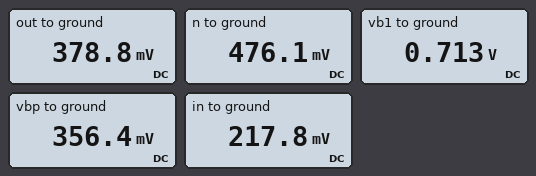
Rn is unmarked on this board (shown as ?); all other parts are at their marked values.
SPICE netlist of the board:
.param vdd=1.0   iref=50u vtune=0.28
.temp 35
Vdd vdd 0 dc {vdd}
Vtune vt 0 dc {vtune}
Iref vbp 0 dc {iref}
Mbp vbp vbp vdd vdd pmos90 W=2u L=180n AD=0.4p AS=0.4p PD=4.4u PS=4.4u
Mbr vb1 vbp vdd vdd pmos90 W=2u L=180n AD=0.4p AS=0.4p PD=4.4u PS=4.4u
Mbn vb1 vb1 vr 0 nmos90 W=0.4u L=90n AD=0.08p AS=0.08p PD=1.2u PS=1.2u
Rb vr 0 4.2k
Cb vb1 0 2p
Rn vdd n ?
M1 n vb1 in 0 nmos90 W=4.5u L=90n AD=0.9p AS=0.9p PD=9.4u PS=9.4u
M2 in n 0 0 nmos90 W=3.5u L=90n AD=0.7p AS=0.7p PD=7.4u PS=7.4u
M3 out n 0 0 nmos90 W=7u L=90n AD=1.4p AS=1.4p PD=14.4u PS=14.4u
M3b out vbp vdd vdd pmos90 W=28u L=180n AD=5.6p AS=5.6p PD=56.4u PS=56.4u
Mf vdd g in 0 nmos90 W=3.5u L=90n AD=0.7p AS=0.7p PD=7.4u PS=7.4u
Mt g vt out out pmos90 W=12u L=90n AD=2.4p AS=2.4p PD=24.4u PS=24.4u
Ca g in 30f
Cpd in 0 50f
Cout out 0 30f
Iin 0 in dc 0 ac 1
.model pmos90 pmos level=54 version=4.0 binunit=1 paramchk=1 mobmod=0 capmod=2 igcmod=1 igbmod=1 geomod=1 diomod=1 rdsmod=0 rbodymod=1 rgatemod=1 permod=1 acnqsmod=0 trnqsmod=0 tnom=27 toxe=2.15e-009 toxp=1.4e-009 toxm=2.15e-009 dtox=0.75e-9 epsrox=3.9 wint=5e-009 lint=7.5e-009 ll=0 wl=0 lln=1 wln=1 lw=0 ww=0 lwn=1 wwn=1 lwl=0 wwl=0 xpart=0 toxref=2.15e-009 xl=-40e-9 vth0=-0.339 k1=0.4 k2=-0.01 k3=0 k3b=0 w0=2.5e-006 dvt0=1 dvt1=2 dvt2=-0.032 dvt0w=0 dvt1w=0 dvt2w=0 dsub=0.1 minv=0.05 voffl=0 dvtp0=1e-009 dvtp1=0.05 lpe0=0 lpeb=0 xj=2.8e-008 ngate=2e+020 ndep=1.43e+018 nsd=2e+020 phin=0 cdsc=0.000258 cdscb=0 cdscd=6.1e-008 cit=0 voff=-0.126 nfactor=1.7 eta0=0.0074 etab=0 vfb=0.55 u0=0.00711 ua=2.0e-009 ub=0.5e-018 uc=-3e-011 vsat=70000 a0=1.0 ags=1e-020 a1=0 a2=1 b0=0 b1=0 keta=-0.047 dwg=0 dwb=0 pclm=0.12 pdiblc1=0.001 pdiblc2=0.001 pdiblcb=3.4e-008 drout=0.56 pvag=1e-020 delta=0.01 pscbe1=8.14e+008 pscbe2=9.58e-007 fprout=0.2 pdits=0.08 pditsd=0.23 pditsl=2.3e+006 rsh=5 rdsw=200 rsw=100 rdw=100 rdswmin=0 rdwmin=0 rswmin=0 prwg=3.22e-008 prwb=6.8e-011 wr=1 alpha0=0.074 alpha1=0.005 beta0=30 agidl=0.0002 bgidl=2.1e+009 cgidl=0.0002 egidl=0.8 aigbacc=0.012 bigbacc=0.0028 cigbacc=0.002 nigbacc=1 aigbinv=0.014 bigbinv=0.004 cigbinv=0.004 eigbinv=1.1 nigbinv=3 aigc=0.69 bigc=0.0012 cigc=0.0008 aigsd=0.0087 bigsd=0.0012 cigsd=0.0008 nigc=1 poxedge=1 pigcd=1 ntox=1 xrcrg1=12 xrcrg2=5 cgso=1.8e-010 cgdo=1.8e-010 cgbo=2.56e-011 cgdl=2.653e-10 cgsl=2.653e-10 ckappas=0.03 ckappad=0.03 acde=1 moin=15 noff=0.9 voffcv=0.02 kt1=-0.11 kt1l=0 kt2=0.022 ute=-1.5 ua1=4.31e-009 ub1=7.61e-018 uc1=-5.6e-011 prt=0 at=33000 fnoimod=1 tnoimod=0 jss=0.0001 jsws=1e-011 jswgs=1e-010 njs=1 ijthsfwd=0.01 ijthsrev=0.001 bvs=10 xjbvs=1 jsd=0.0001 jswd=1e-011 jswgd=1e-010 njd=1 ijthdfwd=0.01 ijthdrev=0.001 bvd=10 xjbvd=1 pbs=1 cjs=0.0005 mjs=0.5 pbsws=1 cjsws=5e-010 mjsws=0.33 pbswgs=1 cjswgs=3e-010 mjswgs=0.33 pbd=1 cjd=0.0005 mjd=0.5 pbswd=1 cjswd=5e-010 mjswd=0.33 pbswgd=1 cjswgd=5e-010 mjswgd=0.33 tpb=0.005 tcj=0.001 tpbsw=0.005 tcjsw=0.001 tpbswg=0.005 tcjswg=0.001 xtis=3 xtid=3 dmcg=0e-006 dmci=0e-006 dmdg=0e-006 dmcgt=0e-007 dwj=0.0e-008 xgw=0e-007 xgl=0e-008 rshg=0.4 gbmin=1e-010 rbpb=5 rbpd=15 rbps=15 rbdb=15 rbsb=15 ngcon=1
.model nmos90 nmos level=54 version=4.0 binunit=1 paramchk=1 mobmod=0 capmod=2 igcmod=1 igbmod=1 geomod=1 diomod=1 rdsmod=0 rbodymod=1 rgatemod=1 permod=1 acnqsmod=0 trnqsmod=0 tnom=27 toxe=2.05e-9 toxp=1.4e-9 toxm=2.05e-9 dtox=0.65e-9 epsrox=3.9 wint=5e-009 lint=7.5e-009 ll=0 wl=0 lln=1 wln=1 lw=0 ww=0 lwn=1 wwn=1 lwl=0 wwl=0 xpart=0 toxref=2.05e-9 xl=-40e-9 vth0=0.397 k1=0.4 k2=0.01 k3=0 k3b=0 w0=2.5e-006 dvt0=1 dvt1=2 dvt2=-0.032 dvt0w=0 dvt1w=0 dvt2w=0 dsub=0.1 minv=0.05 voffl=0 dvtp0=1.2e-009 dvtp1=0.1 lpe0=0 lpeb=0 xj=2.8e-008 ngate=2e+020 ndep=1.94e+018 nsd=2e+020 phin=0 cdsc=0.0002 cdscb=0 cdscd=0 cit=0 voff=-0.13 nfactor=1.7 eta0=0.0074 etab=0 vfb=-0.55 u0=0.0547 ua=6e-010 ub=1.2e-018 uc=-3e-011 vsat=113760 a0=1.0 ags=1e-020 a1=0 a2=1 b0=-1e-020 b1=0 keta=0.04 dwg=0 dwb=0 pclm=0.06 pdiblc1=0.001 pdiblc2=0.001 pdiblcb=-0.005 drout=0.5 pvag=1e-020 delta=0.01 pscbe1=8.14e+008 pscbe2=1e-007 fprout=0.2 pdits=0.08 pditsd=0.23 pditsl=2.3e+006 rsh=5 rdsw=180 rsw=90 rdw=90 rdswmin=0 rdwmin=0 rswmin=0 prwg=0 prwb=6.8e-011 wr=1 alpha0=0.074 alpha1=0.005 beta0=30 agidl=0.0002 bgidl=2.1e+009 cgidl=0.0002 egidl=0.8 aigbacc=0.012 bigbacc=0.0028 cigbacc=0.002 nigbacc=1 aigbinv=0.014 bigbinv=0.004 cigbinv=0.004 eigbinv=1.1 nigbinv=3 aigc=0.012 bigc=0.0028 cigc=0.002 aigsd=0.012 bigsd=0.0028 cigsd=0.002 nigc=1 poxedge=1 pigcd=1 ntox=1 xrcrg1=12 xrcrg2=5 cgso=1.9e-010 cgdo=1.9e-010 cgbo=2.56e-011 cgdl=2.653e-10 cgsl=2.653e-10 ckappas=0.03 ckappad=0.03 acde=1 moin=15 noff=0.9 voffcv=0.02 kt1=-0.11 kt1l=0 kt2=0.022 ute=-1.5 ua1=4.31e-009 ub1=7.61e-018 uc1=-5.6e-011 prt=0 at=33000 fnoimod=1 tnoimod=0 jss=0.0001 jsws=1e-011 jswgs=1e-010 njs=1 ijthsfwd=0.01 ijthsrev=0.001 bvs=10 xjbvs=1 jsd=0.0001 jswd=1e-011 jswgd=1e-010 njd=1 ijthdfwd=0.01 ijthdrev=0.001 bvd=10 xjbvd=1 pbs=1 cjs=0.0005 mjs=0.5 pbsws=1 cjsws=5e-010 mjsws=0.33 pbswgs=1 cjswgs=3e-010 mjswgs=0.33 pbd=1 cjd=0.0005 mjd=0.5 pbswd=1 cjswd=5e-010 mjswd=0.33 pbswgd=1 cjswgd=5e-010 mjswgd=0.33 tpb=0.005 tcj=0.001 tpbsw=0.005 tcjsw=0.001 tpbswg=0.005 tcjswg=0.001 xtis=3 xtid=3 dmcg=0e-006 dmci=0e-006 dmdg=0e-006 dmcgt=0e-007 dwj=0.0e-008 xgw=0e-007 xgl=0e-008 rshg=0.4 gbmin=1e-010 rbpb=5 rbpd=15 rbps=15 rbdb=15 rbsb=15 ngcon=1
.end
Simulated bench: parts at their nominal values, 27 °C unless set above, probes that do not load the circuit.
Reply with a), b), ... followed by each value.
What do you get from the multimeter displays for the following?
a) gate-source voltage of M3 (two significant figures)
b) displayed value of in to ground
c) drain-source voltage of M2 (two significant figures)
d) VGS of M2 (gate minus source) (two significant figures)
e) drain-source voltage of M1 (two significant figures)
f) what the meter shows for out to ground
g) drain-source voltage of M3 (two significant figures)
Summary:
a) 480 mV
b) 217.8 mV
c) 220 mV
d) 480 mV
e) 260 mV
f) 378.8 mV
g) 380 mV
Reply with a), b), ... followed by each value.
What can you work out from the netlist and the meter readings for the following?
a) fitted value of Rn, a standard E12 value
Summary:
a) 1.8 kΩ
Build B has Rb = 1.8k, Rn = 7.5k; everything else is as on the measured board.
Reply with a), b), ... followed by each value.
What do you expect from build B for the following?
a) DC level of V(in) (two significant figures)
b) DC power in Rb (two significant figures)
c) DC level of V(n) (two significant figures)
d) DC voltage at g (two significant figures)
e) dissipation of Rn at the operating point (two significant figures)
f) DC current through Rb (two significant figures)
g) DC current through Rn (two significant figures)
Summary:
a) 200 mV
b) 4.2 µW
c) 450 mV
d) 590 mV
e) 40 µW
f) 48 µA
g) 73 µA
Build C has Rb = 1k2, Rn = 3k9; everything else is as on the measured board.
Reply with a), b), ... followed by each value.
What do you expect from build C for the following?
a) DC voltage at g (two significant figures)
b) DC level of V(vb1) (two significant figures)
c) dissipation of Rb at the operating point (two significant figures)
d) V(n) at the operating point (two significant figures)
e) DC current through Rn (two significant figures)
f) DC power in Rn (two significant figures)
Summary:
a) 490 mV
b) 560 mV
c) 2.8 µW
d) 460 mV
e) 140 µA
f) 74 µW
